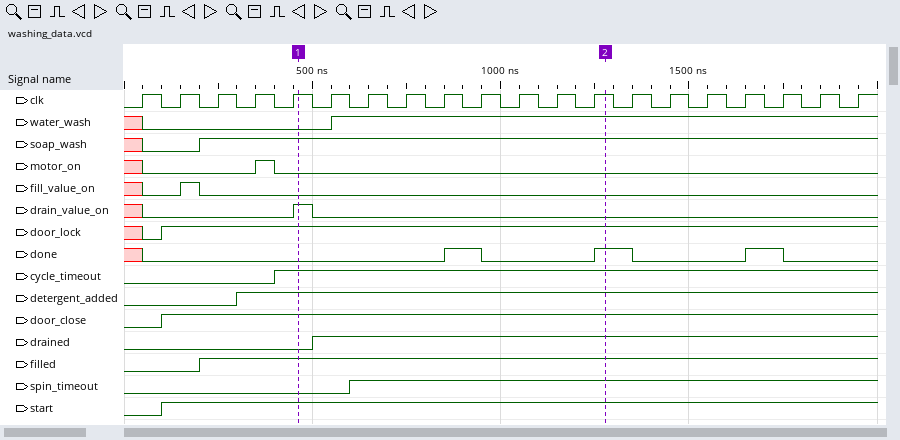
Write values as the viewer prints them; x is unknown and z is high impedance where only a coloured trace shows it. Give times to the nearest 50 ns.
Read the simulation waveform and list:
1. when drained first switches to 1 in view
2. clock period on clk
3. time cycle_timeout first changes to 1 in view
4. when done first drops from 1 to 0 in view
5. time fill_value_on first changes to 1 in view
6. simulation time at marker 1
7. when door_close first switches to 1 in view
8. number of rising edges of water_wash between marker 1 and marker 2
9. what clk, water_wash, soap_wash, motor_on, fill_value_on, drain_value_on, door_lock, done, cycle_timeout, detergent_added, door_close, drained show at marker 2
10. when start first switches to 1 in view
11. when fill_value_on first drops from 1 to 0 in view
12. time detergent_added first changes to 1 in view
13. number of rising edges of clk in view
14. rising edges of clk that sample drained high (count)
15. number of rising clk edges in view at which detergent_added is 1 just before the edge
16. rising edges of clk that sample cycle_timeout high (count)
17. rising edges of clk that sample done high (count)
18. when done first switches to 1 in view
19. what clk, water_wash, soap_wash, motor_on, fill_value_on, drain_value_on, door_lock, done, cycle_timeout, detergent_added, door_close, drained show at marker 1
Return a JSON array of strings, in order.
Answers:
["500 ns", "100 ns", "400 ns", "950 ns", "150 ns", "450 ns", "100 ns", "1", "clk=1, water_wash=1, soap_wash=1, motor_on=0, fill_value_on=0, drain_value_on=0, door_lock=1, done=1, cycle_timeout=1, detergent_added=1, door_close=1, drained=1", "100 ns", "200 ns", "300 ns", "20", "15", "17", "16", "3", "850 ns", "clk=1, water_wash=0, soap_wash=1, motor_on=0, fill_value_on=0, drain_value_on=1, door_lock=1, done=0, cycle_timeout=1, detergent_added=1, door_close=1, drained=0"]
